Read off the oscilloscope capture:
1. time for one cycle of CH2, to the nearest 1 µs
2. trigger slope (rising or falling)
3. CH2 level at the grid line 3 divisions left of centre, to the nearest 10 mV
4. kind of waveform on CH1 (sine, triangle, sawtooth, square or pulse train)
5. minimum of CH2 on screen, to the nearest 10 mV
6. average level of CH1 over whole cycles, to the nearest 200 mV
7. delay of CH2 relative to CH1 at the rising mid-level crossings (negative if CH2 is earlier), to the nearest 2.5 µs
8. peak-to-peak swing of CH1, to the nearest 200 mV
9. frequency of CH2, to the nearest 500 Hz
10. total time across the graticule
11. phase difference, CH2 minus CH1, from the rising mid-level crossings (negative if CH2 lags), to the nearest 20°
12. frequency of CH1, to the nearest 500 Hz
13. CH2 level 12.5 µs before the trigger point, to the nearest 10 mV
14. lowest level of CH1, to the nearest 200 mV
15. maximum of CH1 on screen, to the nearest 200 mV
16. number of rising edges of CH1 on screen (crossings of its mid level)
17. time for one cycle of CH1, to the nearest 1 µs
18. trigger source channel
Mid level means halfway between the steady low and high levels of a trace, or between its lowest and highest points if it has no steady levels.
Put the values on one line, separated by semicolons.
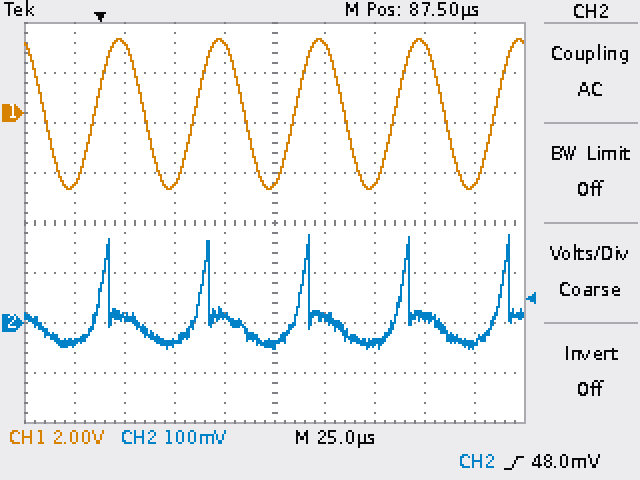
50 µs; rising; 10 mV; sine; -50 mV; 0.0 V; +2.5 µs; 6.0 V; 20.0 kHz; 250 µs; -20°; 20.0 kHz; -40 mV; -3.0 V; 3.0 V; 5; 50 µs; CH2
